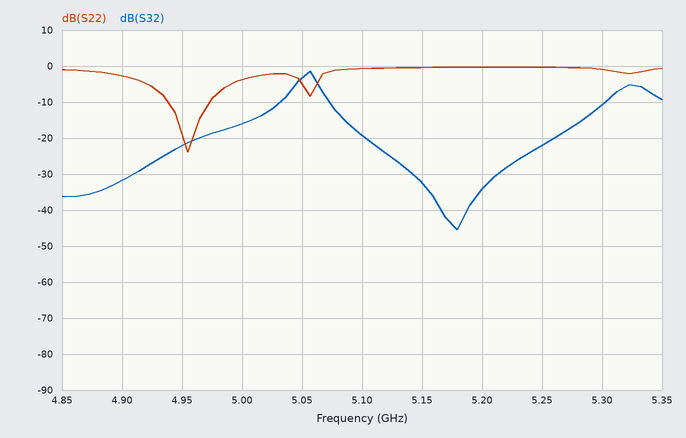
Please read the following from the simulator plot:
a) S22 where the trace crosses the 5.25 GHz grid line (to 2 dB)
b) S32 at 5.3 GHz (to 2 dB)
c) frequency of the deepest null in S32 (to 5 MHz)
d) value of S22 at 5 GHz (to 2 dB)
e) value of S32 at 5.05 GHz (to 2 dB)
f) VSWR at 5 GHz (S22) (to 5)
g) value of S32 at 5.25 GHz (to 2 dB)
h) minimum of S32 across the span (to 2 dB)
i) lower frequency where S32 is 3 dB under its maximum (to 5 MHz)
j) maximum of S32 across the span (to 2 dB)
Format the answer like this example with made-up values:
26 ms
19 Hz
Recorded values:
0 dB
-10 dB
5.180 GHz
-4 dB
-4 dB
5
-22 dB
-46 dB
5.045 GHz
-2 dB
